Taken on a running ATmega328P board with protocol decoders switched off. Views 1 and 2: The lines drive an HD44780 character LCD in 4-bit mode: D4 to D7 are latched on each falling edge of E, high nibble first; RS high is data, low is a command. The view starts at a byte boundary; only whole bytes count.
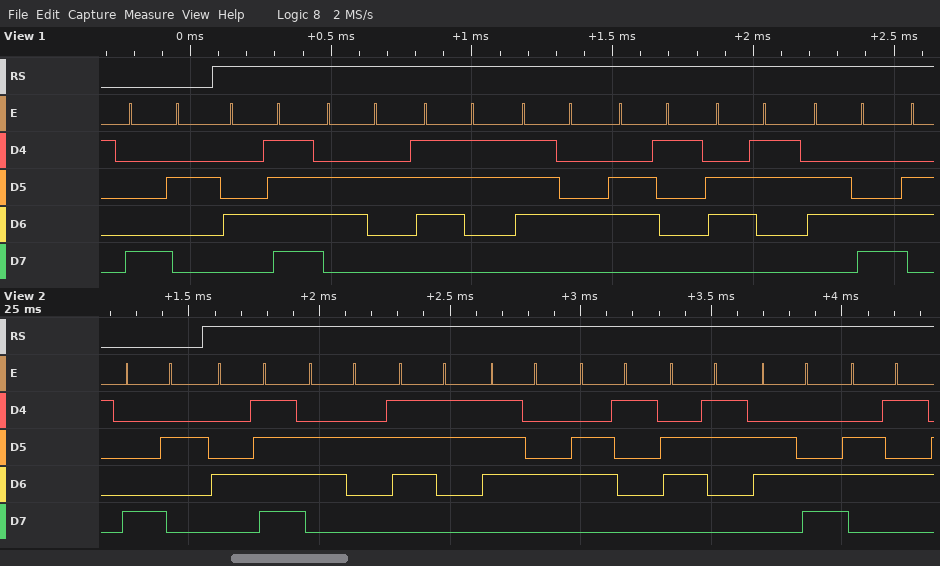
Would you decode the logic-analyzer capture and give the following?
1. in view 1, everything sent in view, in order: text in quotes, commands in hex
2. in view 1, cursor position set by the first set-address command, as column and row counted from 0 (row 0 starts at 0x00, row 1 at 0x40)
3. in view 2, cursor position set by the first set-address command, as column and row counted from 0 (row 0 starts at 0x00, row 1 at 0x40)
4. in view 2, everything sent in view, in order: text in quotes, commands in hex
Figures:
0x82 "Obstacl"
column 2, row 0
column 2, row 0
0x82 "Obstacle"
